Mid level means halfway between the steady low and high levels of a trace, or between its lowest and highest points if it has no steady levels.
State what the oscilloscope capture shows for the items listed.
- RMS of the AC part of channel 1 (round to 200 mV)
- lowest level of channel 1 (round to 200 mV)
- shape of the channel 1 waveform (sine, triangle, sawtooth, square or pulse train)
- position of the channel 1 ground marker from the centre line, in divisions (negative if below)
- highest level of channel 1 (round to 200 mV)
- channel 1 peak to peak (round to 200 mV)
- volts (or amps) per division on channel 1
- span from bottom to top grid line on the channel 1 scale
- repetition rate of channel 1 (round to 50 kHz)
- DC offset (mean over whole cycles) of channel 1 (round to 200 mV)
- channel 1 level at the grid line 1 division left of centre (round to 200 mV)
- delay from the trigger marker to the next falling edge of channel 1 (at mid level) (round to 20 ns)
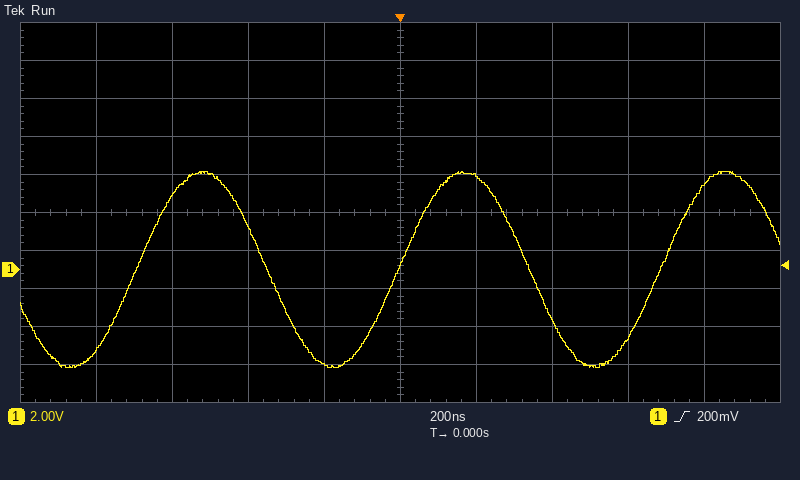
3.6 V
-5.2 V
sine
-1.5 div
5.2 V
10.4 V
2 V
20 V
1.45 MHz
0.0 V
-5.0 V
340 ns
